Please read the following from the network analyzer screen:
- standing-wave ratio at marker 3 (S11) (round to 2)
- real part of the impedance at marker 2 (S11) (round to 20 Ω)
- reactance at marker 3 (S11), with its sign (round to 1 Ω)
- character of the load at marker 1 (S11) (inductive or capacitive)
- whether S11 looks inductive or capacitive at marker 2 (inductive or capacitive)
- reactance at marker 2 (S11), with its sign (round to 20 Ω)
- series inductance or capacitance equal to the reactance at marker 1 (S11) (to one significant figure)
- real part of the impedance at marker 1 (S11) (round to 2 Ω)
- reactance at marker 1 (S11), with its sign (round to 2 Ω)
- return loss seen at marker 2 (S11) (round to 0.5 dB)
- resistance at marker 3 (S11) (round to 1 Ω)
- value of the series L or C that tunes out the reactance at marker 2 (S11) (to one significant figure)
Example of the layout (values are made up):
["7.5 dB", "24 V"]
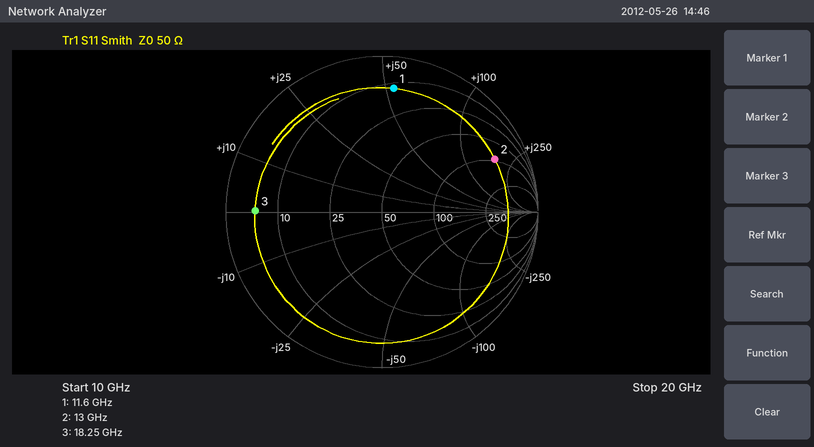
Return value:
["10", "100 Ω", "0 Ω", "inductive", "inductive", "+180 Ω", "700 pH", "12 Ω", "+54 Ω", "2.0 dB", "5 Ω", "70 fF"]
